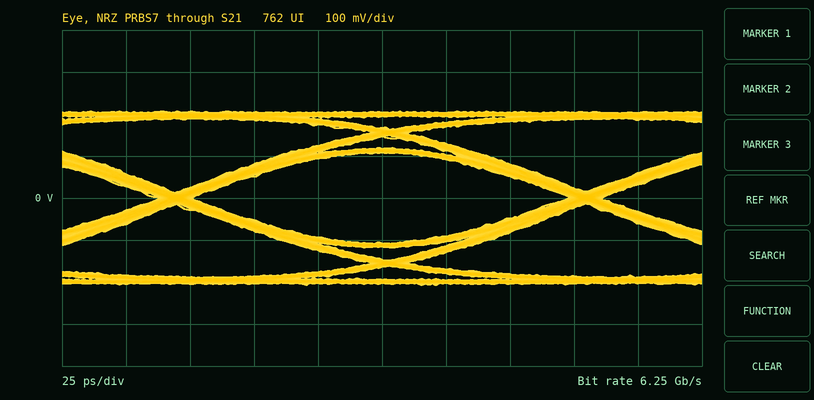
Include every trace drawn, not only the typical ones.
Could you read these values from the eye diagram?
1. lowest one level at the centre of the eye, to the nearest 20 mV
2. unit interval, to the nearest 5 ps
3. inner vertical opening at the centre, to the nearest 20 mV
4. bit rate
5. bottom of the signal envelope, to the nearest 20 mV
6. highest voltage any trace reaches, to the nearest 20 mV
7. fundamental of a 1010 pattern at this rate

100 mV
160 ps
220 mV
6.25 Gb/s
-200 mV
200 mV
3.125 GHz
